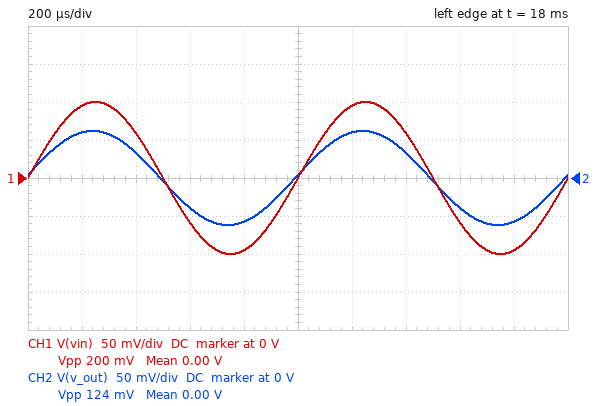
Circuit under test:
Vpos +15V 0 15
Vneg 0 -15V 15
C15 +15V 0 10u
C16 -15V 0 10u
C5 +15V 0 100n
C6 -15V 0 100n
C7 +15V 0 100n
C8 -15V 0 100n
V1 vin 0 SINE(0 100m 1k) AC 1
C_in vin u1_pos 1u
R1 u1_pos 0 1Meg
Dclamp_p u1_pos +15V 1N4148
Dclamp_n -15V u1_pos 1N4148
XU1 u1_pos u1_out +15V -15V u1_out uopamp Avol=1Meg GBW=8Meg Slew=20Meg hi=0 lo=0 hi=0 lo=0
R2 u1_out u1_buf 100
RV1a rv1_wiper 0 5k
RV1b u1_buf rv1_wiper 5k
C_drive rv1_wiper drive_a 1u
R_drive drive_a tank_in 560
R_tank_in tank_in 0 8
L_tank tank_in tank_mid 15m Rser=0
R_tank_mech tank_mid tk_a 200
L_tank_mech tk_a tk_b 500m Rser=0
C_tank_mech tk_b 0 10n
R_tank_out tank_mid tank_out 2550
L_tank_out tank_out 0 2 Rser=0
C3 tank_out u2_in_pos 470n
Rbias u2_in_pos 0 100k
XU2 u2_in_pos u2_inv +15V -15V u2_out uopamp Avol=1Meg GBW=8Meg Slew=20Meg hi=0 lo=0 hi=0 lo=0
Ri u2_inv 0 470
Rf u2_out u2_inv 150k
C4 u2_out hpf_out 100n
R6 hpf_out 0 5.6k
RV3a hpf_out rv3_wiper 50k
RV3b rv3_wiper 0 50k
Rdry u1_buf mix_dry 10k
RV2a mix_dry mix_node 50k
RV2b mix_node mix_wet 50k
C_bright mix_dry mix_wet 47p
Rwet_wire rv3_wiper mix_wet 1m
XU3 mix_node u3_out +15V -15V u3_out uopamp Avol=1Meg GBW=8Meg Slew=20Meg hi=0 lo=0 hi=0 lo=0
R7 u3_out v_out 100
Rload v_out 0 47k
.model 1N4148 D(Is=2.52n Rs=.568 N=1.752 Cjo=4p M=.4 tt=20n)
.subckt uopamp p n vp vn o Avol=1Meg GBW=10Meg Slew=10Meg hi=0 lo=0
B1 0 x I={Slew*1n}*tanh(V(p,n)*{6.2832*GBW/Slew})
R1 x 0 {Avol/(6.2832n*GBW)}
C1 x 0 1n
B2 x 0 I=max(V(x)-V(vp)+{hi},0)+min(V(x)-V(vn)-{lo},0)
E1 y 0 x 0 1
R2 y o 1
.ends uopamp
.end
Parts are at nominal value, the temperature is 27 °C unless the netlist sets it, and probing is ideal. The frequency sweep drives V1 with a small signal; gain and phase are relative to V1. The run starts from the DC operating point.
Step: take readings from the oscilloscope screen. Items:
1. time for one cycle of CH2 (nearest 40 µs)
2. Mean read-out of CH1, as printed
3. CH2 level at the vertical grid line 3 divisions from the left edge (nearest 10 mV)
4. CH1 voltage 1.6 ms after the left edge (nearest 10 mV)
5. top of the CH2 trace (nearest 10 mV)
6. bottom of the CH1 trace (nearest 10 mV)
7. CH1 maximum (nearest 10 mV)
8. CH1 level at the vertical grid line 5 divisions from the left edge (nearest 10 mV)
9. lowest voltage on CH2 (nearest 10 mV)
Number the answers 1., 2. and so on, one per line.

1. 1.00 ms
2. 0.00 V
3. -40 mV
4. -60 mV
5. 60 mV
6. -100 mV
7. 100 mV
8. 0 V
9. -60 mV
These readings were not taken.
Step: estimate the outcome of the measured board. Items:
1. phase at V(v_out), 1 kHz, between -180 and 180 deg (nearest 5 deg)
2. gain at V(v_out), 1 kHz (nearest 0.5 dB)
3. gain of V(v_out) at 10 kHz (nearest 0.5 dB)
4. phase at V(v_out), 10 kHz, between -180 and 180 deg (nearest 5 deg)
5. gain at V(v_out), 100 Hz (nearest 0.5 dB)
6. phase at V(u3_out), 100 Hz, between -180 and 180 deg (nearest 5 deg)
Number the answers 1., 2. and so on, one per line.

1. 5 deg
2. -4.0 dB
3. -4.0 dB
4. 0 deg
5. -5.5 dB
6. 0 deg
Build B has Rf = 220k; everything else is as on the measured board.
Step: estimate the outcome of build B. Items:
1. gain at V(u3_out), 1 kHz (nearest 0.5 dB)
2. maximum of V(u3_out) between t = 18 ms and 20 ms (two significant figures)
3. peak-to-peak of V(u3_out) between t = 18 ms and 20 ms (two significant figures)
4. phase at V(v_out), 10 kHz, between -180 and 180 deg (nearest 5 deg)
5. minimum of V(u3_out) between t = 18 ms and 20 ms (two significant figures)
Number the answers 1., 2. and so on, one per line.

1. -3.5 dB
2. 66 mV
3. 130 mV
4. -5 deg
5. -66 mV
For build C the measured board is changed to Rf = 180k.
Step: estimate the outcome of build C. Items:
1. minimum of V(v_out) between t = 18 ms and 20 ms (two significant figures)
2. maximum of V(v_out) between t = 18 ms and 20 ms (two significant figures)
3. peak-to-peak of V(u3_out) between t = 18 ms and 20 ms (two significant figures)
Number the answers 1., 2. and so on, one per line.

1. -63 mV
2. 63 mV
3. 130 mV
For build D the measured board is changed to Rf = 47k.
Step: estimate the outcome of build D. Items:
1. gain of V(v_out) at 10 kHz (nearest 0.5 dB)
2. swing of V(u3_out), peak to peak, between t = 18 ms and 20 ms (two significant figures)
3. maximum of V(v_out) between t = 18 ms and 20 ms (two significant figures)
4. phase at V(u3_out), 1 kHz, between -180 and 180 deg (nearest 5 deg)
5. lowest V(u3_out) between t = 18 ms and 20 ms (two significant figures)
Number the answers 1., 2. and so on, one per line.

1. -5.0 dB
2. 110 mV
3. 57 mV
4. 0 deg
5. -57 mV
